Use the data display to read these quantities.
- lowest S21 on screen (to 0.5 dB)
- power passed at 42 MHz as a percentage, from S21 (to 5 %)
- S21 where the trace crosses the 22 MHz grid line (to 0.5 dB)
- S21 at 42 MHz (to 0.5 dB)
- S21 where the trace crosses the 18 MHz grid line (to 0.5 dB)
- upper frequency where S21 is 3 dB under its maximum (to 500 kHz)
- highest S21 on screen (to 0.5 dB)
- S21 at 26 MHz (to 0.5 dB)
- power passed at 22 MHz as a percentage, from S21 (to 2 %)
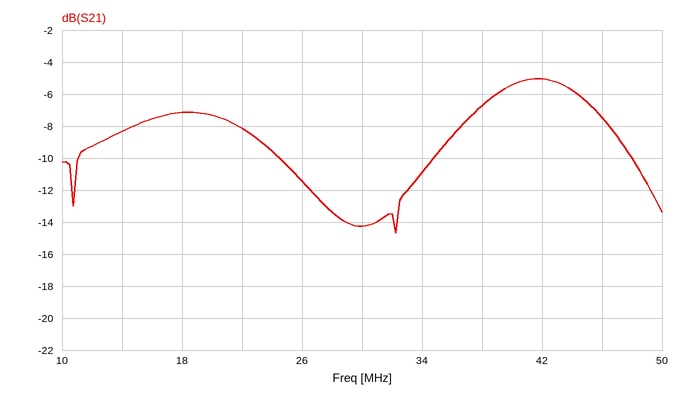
-14.5 dB
30 %
-8.0 dB
-5.0 dB
-7.0 dB
46.5 MHz
-5.0 dB
-11.5 dB
16 %
